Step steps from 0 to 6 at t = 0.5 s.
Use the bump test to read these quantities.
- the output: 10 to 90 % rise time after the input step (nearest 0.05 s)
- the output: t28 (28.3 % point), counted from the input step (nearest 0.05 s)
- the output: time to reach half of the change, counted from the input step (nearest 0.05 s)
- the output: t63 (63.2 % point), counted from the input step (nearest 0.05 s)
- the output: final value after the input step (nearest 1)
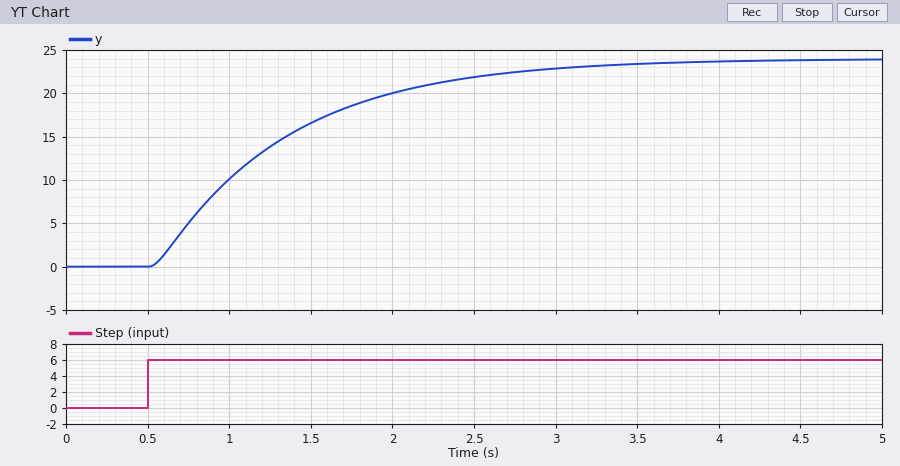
1.75 s
0.35 s
0.60 s
0.85 s
24
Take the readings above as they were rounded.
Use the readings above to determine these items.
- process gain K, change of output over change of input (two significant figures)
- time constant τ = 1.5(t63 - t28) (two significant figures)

4.0
0.75 s
